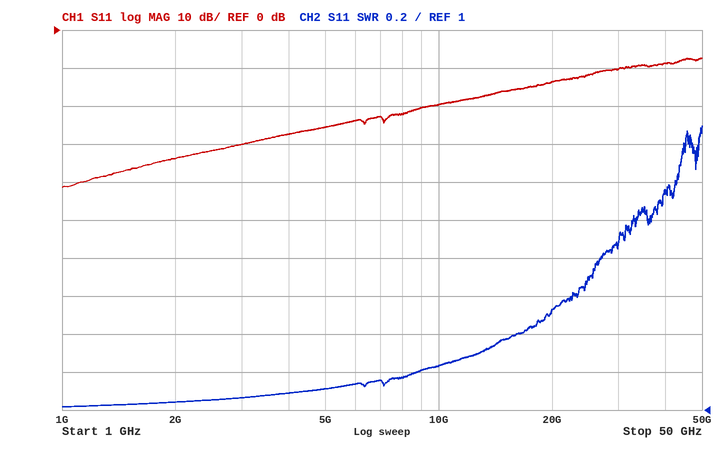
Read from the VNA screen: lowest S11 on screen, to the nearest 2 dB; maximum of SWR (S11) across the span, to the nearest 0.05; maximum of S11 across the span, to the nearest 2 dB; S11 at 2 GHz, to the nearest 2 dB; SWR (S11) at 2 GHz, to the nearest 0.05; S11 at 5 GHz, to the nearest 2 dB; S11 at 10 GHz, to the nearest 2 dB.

-42 dB
2.50
-8 dB
-34 dB
1.05
-26 dB
-20 dB
